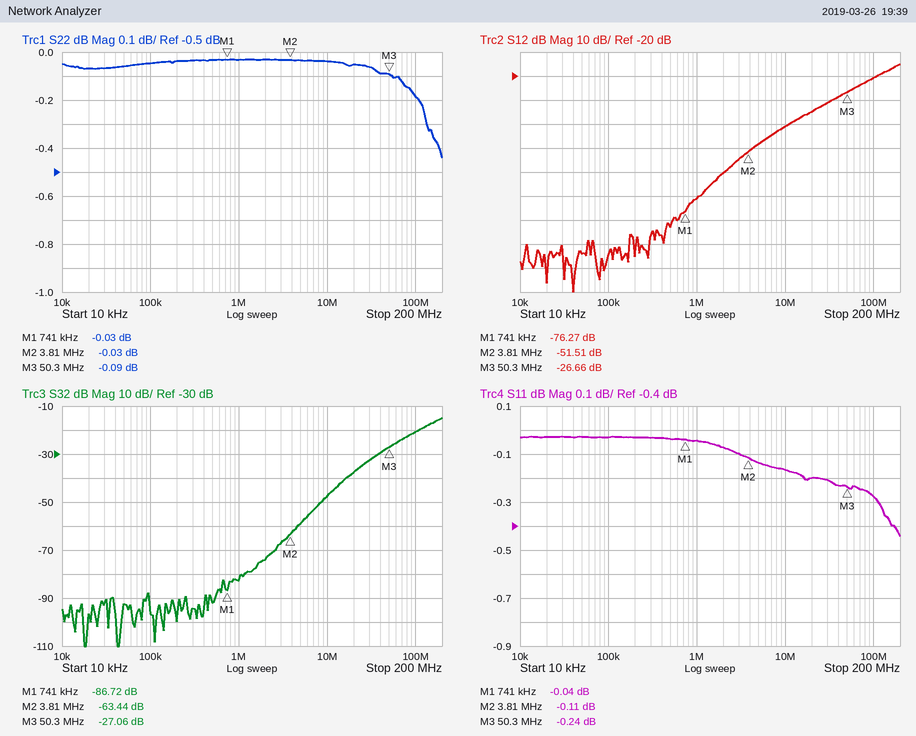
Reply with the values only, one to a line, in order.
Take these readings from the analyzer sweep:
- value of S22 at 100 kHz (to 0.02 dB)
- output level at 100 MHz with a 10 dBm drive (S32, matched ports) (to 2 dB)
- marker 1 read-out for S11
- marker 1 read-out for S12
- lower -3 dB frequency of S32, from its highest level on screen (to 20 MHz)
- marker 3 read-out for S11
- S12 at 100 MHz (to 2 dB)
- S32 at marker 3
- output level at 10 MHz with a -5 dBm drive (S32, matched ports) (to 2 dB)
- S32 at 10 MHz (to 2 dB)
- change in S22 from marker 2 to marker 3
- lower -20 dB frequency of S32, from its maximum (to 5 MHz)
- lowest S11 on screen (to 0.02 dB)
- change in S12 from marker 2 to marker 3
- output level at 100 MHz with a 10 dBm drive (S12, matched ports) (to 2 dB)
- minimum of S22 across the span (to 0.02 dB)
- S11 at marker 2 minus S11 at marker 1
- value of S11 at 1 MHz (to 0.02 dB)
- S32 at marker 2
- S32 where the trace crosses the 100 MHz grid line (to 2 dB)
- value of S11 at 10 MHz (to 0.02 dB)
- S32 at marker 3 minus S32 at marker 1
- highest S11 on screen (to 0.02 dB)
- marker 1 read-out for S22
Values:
-0.04 dB
-10 dBm
-0.04 dB
-76.27 dB
140 MHz
-0.24 dB
-20 dB
-27.06 dB
-52 dBm
-48 dB
-0.06 dB
25 MHz
-0.44 dB
24.85 dB
-10 dBm
-0.44 dB
-0.07 dB
-0.04 dB
-63.44 dB
-20 dB
-0.16 dB
59.66 dB
-0.02 dB
-0.03 dB
